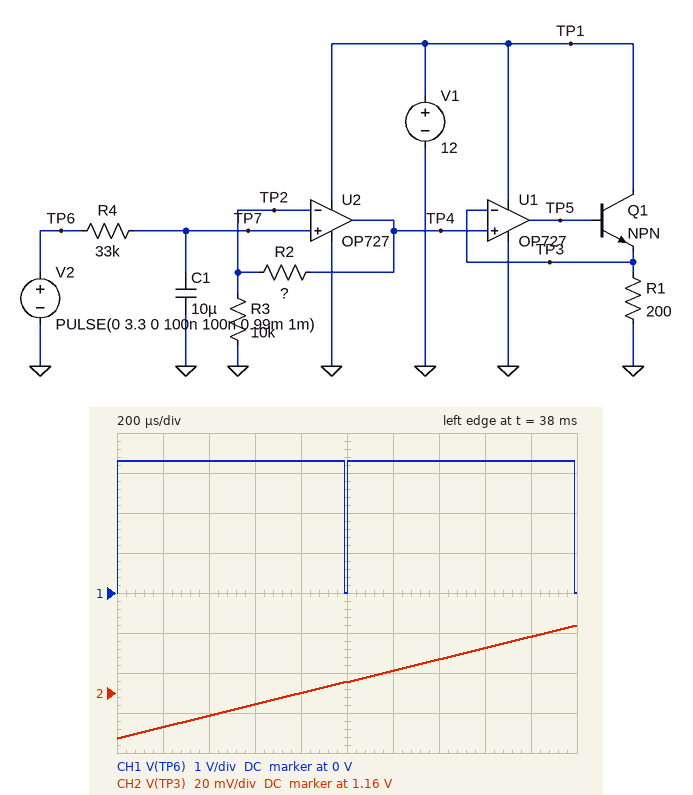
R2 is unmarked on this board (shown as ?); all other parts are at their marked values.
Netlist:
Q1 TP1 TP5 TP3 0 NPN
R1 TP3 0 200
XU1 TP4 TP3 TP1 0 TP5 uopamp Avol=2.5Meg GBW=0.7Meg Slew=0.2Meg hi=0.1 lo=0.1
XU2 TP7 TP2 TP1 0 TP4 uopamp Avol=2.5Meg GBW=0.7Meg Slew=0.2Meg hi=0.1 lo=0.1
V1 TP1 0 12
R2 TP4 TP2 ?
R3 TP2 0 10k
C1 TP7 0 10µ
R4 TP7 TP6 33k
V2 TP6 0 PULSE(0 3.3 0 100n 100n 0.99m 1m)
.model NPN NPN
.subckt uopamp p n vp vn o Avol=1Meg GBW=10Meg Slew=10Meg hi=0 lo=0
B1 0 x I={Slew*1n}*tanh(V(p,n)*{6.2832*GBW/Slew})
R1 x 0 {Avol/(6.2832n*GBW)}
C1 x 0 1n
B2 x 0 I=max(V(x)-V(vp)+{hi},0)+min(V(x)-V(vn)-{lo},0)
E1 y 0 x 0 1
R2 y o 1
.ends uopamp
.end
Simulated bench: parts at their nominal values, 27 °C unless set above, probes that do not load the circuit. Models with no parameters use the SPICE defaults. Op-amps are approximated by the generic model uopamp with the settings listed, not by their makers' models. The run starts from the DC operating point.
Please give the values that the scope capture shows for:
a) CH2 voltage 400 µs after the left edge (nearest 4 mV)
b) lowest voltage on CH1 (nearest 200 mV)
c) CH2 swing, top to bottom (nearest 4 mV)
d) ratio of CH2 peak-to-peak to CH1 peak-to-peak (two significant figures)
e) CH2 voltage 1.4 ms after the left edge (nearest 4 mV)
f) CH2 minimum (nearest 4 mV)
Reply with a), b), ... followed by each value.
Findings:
a) 1.148 V
b) 0 V
c) 56 mV
d) 0.017
e) 1.176 V
f) 1.136 V
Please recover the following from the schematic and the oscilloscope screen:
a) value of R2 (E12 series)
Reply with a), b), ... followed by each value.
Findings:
a) 22 kΩ
